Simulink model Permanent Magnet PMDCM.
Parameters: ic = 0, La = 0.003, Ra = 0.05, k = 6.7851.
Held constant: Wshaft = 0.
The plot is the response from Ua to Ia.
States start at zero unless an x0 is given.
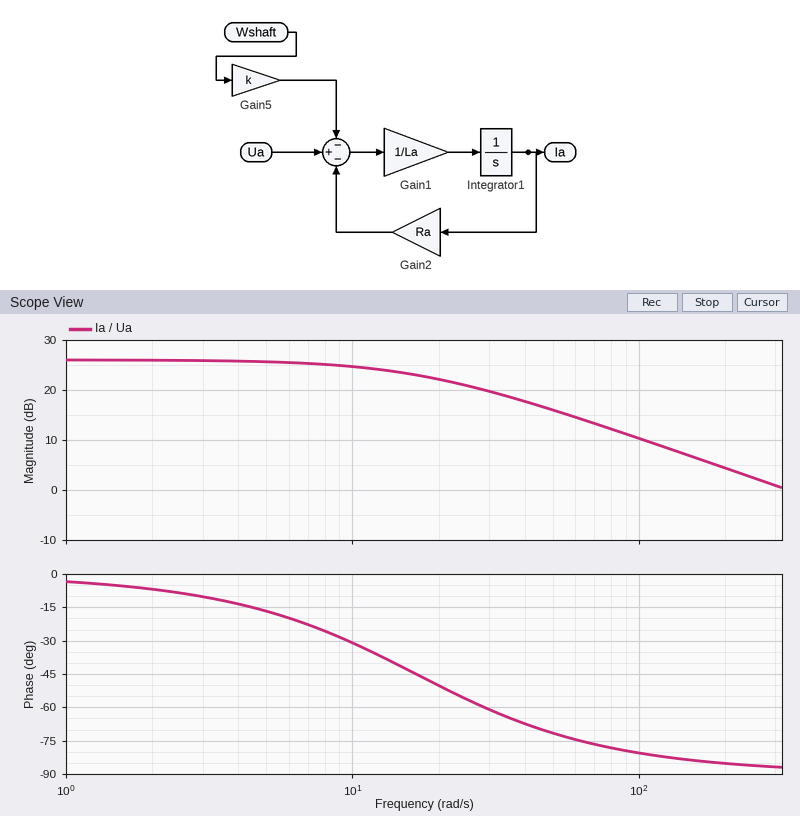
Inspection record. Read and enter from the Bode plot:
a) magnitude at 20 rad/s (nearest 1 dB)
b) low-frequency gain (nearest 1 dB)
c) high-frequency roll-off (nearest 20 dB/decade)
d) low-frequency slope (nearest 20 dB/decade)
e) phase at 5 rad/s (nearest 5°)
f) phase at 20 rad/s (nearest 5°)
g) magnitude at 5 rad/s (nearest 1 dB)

22 dB
26 dB
-20 dB/decade
0 dB/decade
-15°
-50°
26 dB
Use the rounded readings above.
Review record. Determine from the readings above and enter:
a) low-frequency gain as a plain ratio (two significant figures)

20
